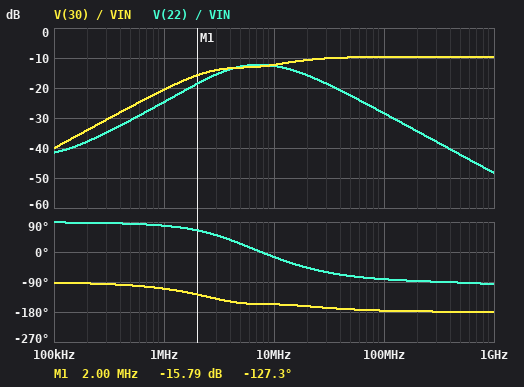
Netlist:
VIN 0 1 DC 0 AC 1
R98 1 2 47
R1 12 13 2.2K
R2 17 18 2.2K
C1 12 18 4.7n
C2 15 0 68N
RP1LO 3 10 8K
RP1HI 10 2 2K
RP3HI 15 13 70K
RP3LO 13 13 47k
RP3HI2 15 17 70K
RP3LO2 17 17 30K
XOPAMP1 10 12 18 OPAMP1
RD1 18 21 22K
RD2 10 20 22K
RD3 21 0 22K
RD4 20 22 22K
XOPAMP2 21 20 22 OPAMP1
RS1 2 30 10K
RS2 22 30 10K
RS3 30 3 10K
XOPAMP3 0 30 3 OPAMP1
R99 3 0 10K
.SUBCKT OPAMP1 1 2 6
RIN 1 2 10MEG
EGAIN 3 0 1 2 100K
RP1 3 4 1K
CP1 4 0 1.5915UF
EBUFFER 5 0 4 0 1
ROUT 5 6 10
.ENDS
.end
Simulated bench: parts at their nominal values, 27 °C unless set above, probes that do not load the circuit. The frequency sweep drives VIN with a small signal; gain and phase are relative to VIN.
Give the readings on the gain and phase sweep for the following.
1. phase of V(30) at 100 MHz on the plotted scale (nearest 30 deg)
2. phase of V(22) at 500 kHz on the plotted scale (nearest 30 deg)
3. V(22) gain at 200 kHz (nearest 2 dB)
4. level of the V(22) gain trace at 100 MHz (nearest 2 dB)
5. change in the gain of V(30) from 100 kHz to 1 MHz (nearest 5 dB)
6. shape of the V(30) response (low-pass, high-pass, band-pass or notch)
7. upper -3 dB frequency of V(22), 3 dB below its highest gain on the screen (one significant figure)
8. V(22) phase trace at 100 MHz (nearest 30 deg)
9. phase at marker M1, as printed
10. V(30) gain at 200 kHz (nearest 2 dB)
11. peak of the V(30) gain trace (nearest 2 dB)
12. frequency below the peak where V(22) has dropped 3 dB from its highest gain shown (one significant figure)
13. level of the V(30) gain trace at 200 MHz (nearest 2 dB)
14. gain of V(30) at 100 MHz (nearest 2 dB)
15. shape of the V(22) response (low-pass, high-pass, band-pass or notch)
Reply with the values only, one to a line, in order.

-180 deg
90 deg
-38 dB
-28 dB
20 dB
high-pass
20 MHz
-90 deg
-127.3 deg
-34 dB
-10 dB
3 MHz
-10 dB
-10 dB
band-pass
